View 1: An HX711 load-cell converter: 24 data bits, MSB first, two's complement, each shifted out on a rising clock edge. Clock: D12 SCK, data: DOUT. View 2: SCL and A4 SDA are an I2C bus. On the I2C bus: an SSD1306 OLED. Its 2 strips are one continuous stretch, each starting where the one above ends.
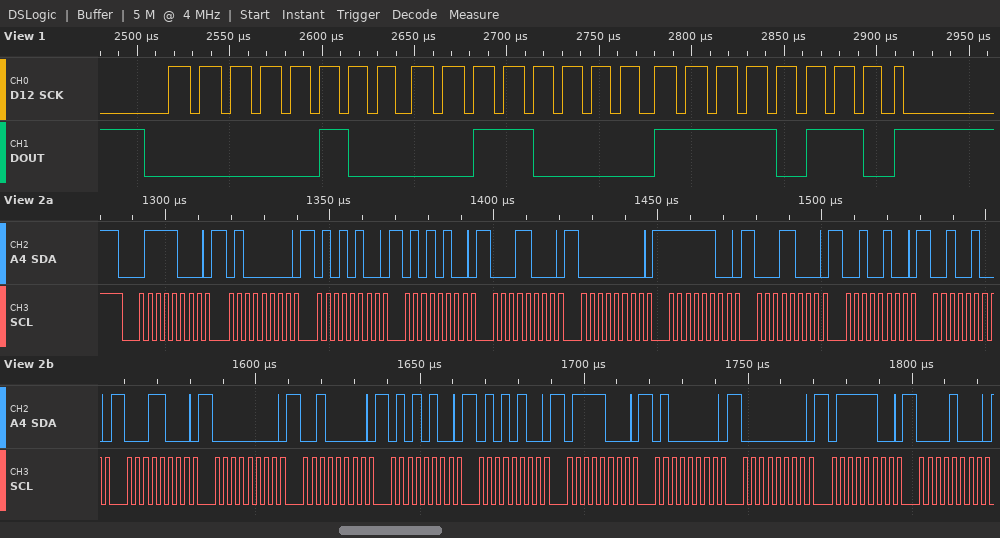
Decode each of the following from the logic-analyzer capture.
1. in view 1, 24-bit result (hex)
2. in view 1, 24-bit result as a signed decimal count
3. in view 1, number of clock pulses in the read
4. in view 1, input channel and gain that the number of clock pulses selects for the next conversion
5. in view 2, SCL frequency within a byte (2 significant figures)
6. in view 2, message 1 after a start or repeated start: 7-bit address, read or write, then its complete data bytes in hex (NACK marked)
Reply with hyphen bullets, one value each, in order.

- 0x0430F6
- 274678
- 25
- channel A, gain 128
- 400 kHz
- 0x3C write: 40 54 54 18 00 FC 18 24 24 18 00 20 54 54 78 40 00 7C 08
